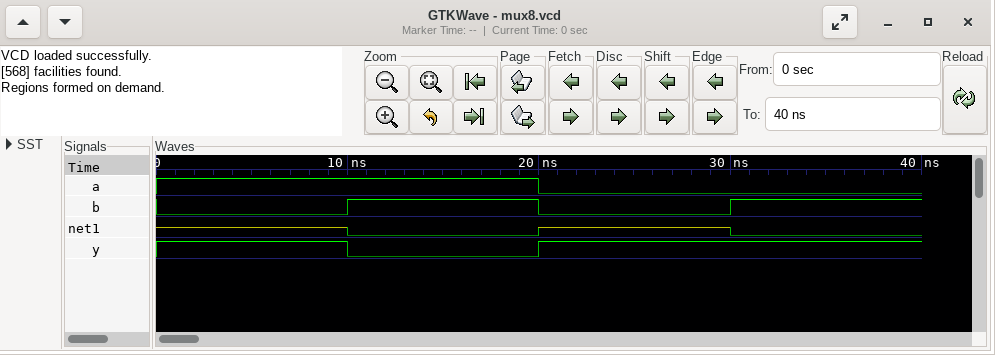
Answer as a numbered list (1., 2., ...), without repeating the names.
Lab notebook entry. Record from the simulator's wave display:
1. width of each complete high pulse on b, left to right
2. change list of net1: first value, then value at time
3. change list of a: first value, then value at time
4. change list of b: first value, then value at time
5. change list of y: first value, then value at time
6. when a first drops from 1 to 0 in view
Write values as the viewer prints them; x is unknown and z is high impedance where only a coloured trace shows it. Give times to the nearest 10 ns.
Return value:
1. 10 ns
2. z, 0 at 10 ns, z at 20 ns, 0 at 30 ns
3. 1, 0 at 20 ns
4. 0, 1 at 10 ns, 0 at 20 ns, 1 at 30 ns
5. 1, 0 at 10 ns, 1 at 20 ns
6. 20 ns
